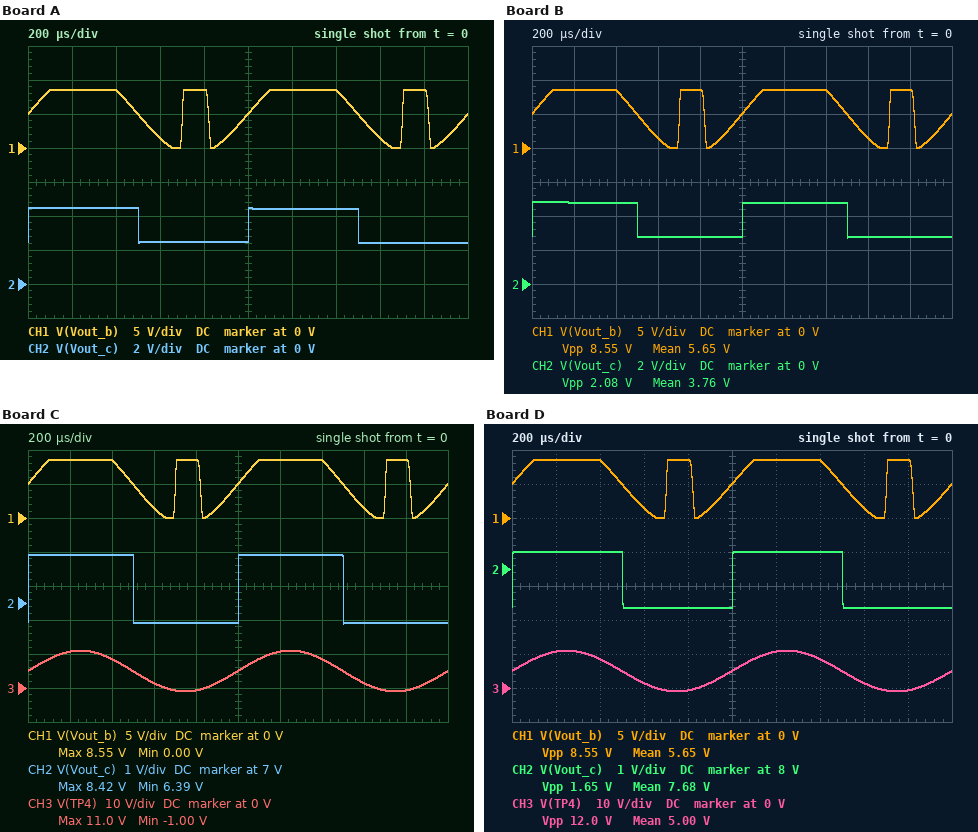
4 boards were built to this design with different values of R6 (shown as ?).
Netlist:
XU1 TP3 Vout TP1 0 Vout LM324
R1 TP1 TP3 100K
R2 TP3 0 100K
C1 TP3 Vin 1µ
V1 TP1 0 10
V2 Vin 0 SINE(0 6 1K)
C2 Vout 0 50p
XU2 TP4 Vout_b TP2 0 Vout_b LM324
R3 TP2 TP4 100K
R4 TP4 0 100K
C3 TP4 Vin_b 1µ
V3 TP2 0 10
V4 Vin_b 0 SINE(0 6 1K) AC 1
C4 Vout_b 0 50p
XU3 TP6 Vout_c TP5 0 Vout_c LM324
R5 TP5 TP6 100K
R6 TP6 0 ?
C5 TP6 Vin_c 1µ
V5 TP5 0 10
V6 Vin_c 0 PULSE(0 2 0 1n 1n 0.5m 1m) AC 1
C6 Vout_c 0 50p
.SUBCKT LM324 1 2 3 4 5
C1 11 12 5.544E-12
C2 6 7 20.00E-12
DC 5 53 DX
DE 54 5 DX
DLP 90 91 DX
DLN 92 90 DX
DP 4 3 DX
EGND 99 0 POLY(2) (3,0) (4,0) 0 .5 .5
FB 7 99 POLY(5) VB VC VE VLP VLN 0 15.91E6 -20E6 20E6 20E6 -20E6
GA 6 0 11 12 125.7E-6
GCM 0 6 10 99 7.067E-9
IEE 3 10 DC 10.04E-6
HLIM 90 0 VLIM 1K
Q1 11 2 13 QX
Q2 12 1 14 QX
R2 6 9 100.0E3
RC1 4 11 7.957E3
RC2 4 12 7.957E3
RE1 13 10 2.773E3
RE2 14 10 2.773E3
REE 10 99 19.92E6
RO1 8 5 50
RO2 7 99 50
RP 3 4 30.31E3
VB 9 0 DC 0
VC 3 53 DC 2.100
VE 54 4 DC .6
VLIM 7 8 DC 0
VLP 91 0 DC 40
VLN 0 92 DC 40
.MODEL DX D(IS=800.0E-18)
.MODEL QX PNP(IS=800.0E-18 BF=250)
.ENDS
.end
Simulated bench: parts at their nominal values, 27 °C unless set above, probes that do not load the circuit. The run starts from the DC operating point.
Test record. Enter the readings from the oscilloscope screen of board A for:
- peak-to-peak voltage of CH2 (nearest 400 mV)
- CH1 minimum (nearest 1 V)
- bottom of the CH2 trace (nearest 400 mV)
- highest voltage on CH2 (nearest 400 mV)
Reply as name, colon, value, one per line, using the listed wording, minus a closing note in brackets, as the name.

peak-to-peak voltage of CH2: 2.0 V
CH1 minimum: 0 V
bottom of the CH2 trace: 2.4 V
highest voltage on CH2: 4.4 V
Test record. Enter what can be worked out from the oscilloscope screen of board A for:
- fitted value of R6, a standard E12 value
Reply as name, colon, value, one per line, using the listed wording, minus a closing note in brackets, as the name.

fitted value of R6, a standard E12 value: 33 kΩ
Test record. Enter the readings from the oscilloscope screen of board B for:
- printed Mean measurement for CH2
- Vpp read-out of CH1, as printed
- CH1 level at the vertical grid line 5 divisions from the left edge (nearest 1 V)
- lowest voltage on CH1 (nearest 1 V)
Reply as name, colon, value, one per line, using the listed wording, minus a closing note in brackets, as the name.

printed Mean measurement for CH2: 3.76 V
Vpp read-out of CH1, as printed: 8.55 V
CH1 level at the vertical grid line 5 divisions from the left edge: 5 V
lowest voltage on CH1: 0 V
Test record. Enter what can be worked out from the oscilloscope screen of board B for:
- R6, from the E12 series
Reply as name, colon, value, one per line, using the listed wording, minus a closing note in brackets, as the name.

R6, from the E12 series: 39 kΩ
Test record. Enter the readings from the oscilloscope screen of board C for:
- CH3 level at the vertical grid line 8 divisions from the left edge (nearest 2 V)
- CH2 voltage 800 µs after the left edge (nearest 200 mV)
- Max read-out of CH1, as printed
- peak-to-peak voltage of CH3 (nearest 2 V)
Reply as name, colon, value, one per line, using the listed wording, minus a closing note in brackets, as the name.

CH3 level at the vertical grid line 8 divisions from the left edge: 2 V
CH2 voltage 800 µs after the left edge: 6.4 V
Max read-out of CH1, as printed: 8.55 V
peak-to-peak voltage of CH3: 12 V
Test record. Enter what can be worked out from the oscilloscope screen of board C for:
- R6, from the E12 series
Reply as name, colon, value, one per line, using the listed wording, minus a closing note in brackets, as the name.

R6, from the E12 series: 180 kΩ
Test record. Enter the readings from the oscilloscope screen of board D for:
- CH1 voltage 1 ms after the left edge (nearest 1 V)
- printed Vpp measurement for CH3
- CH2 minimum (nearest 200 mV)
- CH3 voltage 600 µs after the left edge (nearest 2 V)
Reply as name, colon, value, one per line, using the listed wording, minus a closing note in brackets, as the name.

CH1 voltage 1 ms after the left edge: 5 V
printed Vpp measurement for CH3: 12.0 V
CH2 minimum: 6.8 V
CH3 voltage 600 µs after the left edge: 2 V
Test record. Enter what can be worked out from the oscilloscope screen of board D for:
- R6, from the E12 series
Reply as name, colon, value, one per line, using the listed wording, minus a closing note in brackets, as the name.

R6, from the E12 series: 220 kΩ
